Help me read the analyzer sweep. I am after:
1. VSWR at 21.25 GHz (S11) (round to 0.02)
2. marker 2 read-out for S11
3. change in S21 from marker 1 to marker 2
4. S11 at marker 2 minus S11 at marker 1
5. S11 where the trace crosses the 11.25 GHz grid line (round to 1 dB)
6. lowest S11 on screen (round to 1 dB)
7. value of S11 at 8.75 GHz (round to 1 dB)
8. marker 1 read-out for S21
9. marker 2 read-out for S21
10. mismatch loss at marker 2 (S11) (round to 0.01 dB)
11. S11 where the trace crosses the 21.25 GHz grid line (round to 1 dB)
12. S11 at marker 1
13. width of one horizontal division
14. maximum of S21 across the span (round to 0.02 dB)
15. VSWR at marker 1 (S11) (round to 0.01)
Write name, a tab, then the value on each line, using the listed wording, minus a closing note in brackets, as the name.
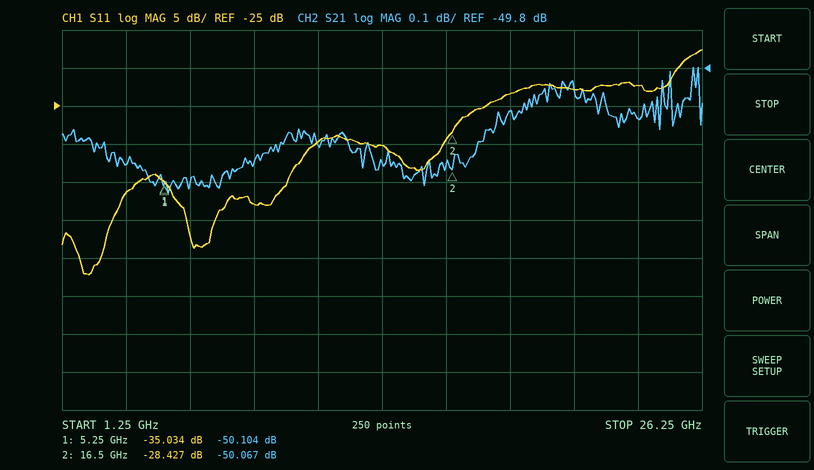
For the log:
VSWR at 21.25 GHz (S11)	1.16
marker 2 read-out for S11	-28.427 dB
change in S21 from marker 1 to marker 2	0.037 dB
S11 at marker 2 minus S11 at marker 1	6.607 dB
S11 where the trace crosses the 11.25 GHz grid line	-30 dB
lowest S11 on screen	-47 dB
value of S11 at 8.75 GHz	-38 dB
marker 1 read-out for S21	-50.104 dB
marker 2 read-out for S21	-50.067 dB
mismatch loss at marker 2 (S11)	0.01 dB
S11 where the trace crosses the 21.25 GHz grid line	-23 dB
S11 at marker 1	-35.034 dB
width of one horizontal division	2.5 GHz
maximum of S21 across the span	-49.80 dB
VSWR at marker 1 (S11)	1.04
